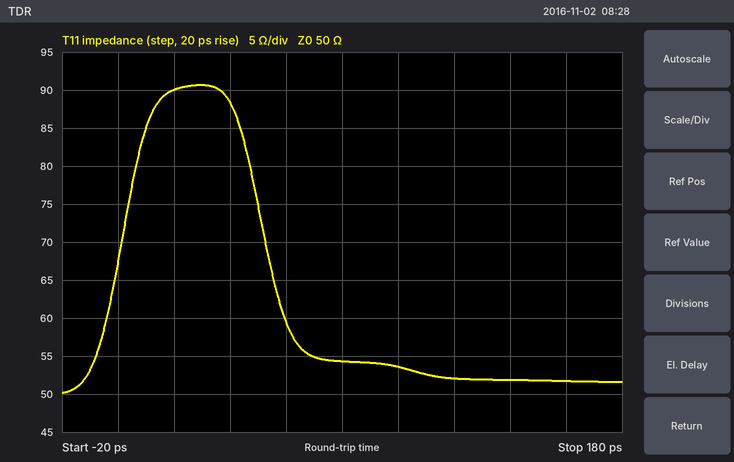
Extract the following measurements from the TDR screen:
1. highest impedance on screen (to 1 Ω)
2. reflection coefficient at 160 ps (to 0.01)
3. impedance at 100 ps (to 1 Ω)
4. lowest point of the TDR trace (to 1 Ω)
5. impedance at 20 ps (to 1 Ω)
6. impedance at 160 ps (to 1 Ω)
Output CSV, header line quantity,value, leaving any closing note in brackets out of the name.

quantity,value
highest impedance on screen,91 Ω
reflection coefficient at 160 ps,+0.02
impedance at 100 ps,54 Ω
lowest point of the TDR trace,50 Ω
impedance at 20 ps,90 Ω
impedance at 160 ps,52 Ω
